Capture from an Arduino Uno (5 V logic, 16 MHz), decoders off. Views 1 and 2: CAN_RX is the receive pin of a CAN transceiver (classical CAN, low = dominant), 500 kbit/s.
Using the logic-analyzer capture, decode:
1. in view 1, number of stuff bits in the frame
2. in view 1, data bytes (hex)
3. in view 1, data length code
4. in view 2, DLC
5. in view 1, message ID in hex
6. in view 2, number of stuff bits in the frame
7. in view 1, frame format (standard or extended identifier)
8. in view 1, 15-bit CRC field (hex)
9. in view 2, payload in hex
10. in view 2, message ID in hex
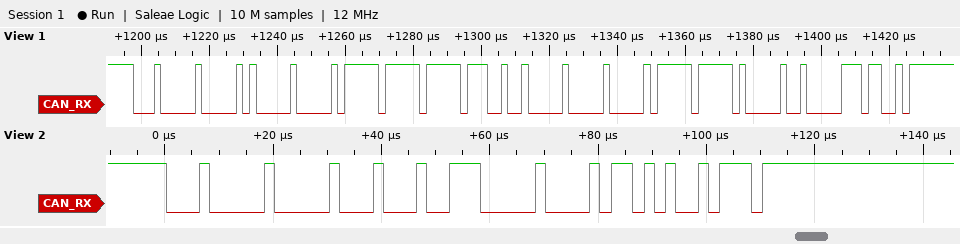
14
00 FF FF C9 00 00 FF E0
8
2
0x100
3
standard
0x106C
27 00
0x100
